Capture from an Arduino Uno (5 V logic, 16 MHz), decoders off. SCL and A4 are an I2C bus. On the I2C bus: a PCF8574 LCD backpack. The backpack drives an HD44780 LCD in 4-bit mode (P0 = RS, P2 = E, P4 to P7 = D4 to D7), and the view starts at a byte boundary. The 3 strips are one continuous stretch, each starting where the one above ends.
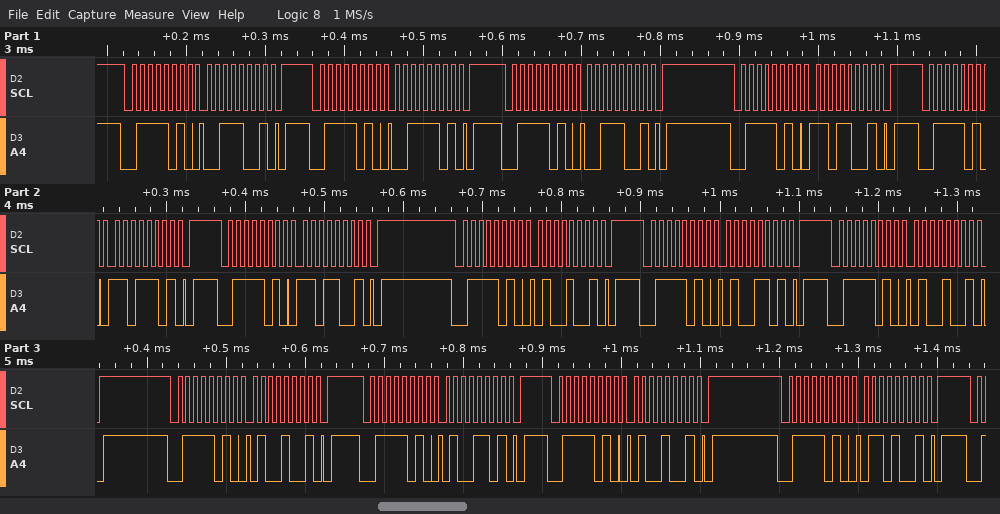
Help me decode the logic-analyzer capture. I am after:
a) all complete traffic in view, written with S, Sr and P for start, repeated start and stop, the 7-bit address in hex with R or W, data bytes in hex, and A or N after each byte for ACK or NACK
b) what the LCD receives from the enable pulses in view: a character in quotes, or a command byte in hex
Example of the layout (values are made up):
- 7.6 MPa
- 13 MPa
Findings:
- S 3DW A 39 A P S 3DW A 3D A P S 3DW A 39 A P S 3DW A D9 A P S 3DW A DD A P S 3DW A D9 A P S 3DW A 49 A P S 3DW A 4D A P S 3DW A 49 A P S 3DW A 49 A P S 3DW A 4D A P S 3DW A 49 A P S 3DW A 69 A P
- '=' 'D'
